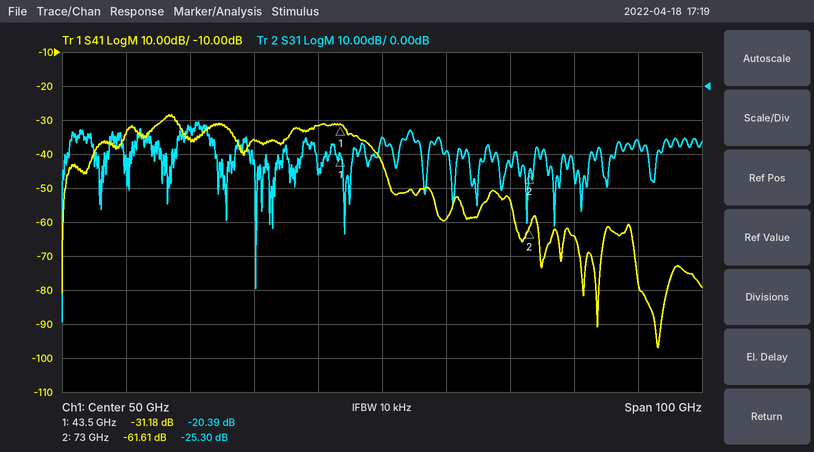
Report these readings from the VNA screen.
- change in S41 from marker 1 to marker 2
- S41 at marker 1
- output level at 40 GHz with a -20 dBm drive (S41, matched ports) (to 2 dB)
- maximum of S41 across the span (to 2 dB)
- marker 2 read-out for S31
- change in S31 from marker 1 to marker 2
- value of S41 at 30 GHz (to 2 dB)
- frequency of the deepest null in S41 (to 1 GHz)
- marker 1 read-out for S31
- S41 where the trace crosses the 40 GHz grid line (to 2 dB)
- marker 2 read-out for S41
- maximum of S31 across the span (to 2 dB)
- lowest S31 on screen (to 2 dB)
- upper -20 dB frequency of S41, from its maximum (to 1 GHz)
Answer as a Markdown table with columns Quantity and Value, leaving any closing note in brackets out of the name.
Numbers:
| Quantity | Value |
|---|---|
| change in S41 from marker 1 to marker 2 | -30.43 dB |
| S41 at marker 1 | -31.18 dB |
| output level at 40 GHz with a -20 dBm drive (S41, matched ports) | -52 dBm |
| maximum of S41 across the span | -28 dB |
| marker 2 read-out for S31 | -25.30 dB |
| change in S31 from marker 1 to marker 2 | -4.91 dB |
| value of S41 at 30 GHz | -36 dB |
| frequency of the deepest null in S41 | 93 GHz |
| marker 1 read-out for S31 | -20.39 dB |
| S41 where the trace crosses the 40 GHz grid line | -32 dB |
| marker 2 read-out for S41 | -61.61 dB |
| maximum of S31 across the span | -10 dB |
| lowest S31 on screen | -70 dB |
| upper -20 dB frequency of S41, from its maximum | 51 GHz |
